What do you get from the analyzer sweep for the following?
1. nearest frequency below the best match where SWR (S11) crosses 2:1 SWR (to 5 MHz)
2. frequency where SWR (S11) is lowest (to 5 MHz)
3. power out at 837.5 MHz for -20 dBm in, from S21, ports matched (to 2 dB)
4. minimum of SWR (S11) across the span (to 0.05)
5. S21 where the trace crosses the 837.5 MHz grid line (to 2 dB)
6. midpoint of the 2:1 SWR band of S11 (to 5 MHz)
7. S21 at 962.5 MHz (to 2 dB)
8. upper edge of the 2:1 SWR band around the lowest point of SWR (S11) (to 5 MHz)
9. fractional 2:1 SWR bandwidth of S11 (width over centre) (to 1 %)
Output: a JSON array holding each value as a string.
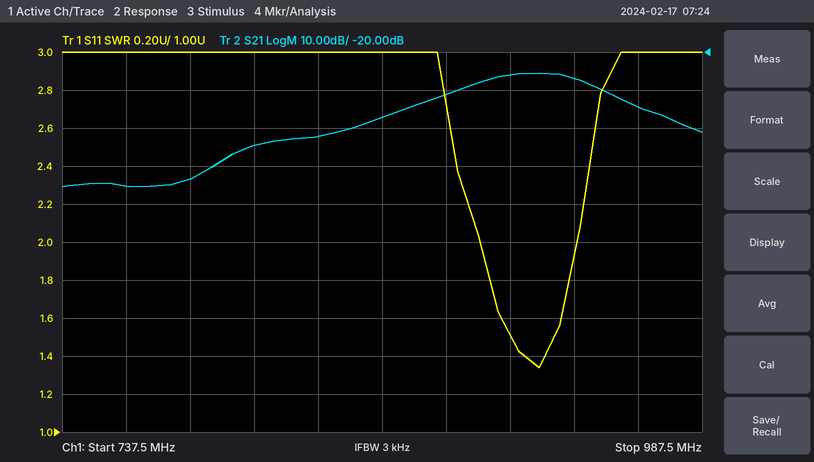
["900 MHz", "925 MHz", "-62 dBm", "1.35", "-42 dB", "920 MHz", "-34 dB", "940 MHz", "4 %"]
